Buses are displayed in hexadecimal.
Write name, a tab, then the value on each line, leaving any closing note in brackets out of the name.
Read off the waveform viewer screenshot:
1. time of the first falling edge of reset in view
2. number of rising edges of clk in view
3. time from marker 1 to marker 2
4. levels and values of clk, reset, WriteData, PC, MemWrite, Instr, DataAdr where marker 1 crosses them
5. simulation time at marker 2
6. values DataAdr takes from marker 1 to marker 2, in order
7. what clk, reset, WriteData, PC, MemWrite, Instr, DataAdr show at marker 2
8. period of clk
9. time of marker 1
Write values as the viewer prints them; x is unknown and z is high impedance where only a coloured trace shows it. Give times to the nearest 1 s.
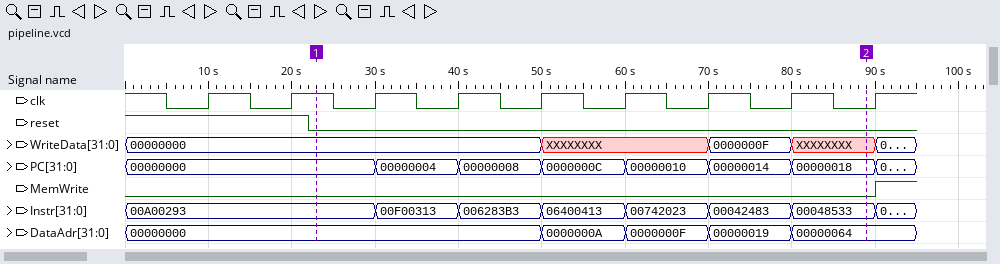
time of the first falling edge of reset in view	22 s
number of rising edges of clk in view	9
time from marker 1 to marker 2	66 s
levels and values of clk, reset, WriteData, PC, MemWrite, Instr, DataAdr where marker 1 crosses them	clk=1, reset=0, WriteData=00000000, PC=00000000, MemWrite=0, Instr=00A00293, DataAdr=00000000
simulation time at marker 2	89 s
values DataAdr takes from marker 1 to marker 2, in order	00000000, 0000000A, 0000000F, 00000019, 00000064
what clk, reset, WriteData, PC, MemWrite, Instr, DataAdr show at marker 2	clk=0, reset=0, WriteData=XXXXXXXX, PC=00000018, MemWrite=0, Instr=00048533, DataAdr=00000064
period of clk	10 s
time of marker 1	23 s
